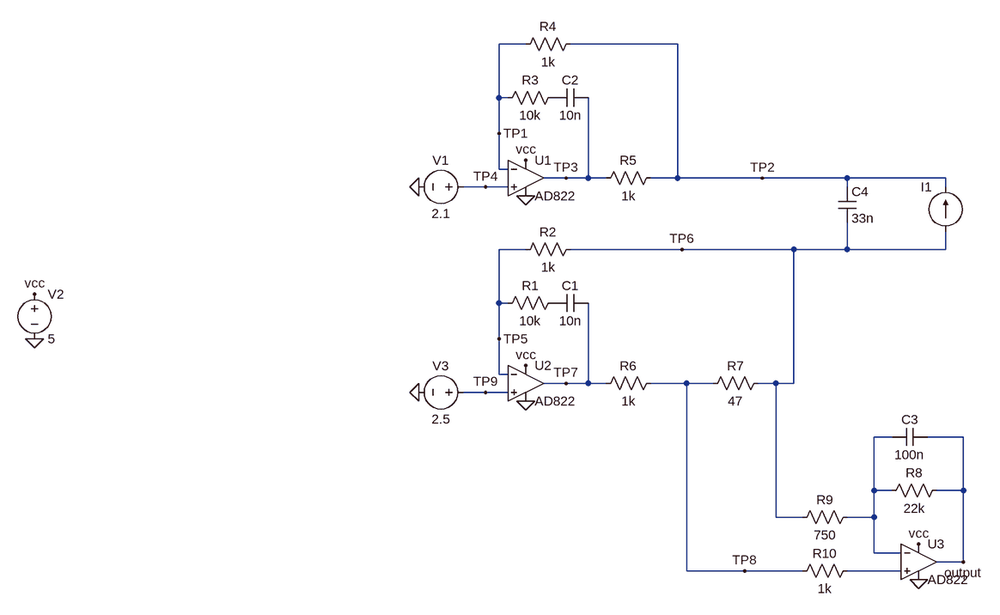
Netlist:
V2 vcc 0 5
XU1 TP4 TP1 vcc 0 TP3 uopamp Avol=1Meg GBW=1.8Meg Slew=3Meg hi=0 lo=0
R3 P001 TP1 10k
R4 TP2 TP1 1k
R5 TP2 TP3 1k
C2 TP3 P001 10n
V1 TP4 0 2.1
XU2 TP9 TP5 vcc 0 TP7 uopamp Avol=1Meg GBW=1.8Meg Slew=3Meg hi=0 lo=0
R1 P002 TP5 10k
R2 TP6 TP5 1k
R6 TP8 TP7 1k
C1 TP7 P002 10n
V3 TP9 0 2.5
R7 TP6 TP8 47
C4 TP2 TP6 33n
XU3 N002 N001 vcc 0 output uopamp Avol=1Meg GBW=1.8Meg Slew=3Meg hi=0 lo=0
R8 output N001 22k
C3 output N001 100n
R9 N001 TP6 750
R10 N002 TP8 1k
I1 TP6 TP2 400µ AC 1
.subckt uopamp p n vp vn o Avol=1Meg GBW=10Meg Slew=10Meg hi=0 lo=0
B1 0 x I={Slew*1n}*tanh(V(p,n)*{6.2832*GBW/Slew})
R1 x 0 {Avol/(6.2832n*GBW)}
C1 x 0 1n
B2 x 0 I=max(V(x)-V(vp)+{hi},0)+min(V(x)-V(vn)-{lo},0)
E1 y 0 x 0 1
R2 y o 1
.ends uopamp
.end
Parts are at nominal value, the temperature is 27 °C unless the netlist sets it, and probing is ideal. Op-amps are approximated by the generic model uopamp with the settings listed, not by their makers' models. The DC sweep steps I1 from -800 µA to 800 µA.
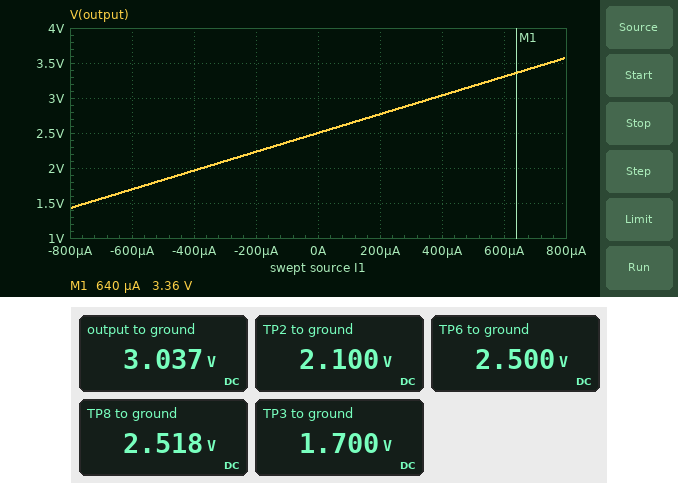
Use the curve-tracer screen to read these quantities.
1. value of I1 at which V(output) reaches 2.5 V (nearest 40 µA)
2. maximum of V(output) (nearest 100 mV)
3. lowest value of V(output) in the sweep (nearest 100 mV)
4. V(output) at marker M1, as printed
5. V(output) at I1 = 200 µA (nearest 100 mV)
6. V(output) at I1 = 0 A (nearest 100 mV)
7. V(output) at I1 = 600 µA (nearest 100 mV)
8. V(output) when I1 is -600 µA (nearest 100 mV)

0 A
3.6 V
1.4 V
3.36 V
2.8 V
2.5 V
3.3 V
1.7 V
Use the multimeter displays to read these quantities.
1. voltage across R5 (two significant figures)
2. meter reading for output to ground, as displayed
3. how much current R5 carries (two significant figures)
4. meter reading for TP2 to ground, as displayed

400 mV
3.037 V
400 µA
2.100 V
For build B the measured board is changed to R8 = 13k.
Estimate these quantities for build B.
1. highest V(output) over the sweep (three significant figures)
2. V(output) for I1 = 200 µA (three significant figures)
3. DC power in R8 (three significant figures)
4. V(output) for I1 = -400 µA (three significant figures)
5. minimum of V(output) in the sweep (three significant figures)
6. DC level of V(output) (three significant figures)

3.15 V
2.66 V
7.23 µW
2.18 V
1.85 V
2.82 V
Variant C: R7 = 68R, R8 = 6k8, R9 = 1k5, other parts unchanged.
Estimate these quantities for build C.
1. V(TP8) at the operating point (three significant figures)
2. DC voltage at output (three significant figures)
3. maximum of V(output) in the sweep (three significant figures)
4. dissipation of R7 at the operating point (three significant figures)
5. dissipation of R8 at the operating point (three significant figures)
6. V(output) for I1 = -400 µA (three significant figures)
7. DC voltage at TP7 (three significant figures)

2.53 V
2.64 V
2.79 V
9.96 µW
2.05 µW
2.36 V
2.91 V
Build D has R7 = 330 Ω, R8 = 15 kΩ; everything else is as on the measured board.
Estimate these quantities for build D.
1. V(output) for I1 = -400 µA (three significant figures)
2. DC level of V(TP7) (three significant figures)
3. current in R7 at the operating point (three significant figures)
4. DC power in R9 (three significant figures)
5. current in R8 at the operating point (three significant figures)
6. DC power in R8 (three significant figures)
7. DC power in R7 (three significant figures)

575 mV
2.87 V
278 µA
11.2 µW
122 µA
224 µW
25.5 µW
